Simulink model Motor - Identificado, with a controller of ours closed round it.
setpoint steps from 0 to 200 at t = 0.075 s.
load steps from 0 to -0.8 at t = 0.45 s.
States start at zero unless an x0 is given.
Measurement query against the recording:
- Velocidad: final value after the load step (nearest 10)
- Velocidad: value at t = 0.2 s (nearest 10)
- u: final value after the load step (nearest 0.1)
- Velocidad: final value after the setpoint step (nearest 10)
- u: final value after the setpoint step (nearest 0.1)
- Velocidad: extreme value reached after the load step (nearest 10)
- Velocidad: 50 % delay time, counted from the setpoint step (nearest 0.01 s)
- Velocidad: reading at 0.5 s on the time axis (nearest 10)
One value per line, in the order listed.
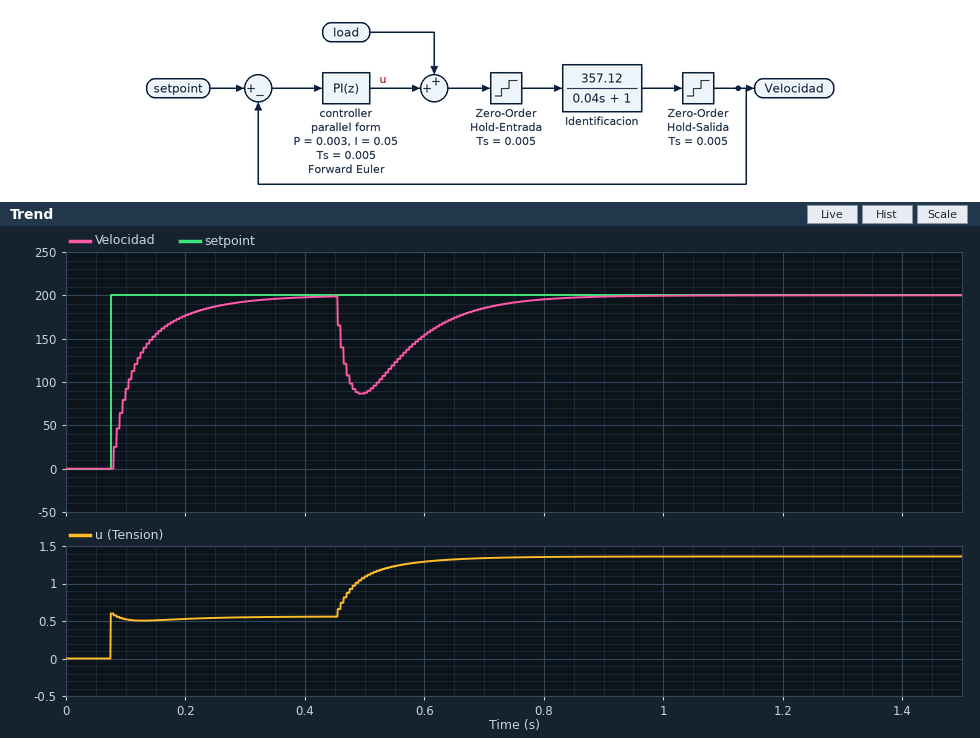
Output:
200
180
1.4
200
0.6
90
0.03 s
90
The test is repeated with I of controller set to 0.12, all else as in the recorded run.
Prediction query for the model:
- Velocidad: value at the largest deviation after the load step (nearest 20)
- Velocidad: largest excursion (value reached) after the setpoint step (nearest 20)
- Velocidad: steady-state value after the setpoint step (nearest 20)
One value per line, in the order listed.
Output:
100
220
200
